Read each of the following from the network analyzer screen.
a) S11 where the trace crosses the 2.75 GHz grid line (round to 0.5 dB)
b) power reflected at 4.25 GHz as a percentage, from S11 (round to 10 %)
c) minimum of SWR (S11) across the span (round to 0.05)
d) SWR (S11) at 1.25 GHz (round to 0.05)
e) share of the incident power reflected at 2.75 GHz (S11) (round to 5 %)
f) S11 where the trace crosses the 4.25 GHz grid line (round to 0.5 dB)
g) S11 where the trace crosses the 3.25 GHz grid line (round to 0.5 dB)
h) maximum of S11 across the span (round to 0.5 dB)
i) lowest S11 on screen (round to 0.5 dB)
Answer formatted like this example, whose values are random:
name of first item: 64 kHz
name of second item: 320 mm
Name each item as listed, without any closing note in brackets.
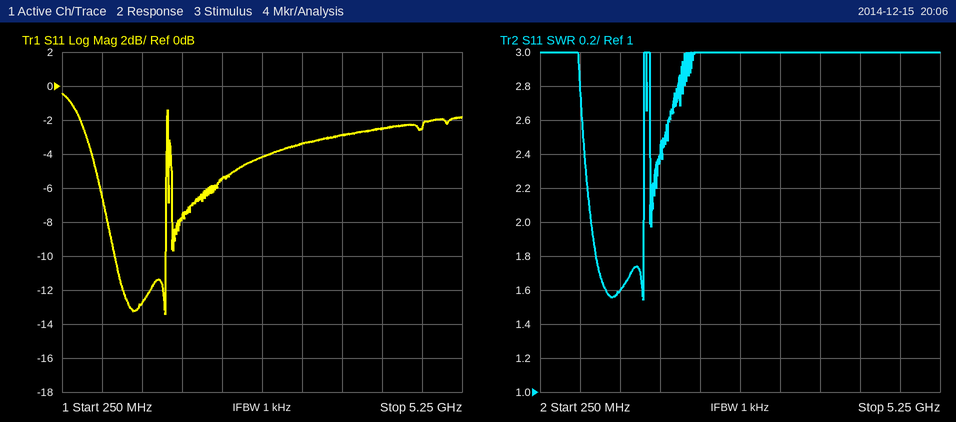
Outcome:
S11 where the trace crosses the 2.75 GHz grid line: -4.0 dB
power reflected at 4.25 GHz as a percentage, from S11: 60 %
minimum of SWR (S11) across the span: 1.55
SWR (S11) at 1.25 GHz: 1.60
share of the incident power reflected at 2.75 GHz (S11): 40 %
S11 where the trace crosses the 4.25 GHz grid line: -2.5 dB
S11 where the trace crosses the 3.25 GHz grid line: -3.5 dB
maximum of S11 across the span: -0.5 dB
lowest S11 on screen: -13.5 dB
